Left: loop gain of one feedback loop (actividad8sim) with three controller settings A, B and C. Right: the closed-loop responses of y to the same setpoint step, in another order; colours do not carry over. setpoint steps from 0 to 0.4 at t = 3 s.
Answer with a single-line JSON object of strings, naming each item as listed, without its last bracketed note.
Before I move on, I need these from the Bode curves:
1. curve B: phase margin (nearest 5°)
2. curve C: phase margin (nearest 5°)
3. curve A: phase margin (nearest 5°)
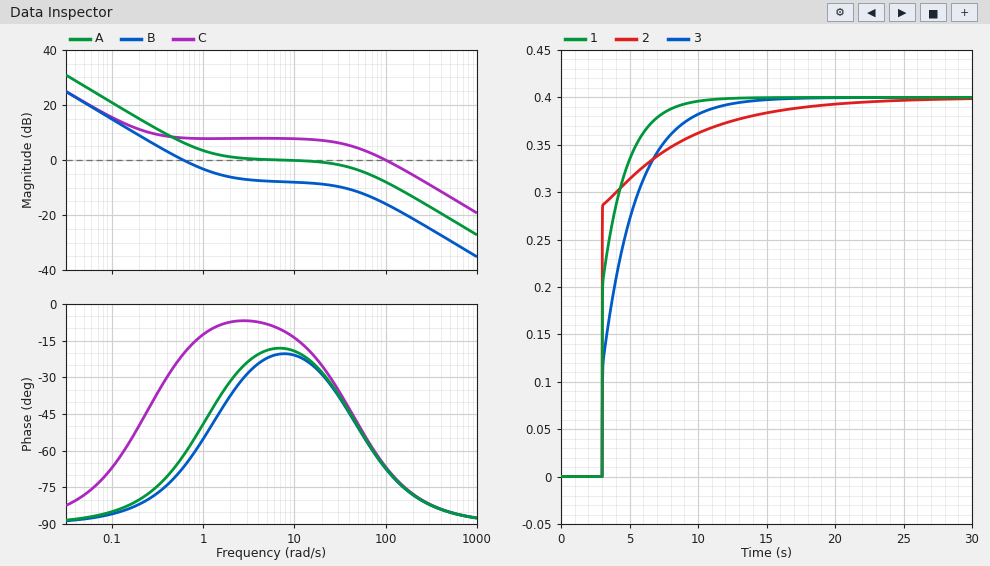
{"curve B: phase margin": "115°", "curve C: phase margin": "115°", "curve A: phase margin": "160°"}
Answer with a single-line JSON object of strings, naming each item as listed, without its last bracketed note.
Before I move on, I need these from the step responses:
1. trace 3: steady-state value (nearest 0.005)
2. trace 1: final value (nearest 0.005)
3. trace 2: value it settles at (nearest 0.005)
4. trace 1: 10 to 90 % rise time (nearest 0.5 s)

{"trace 3: steady-state value": "0.400", "trace 1: final value": "0.400", "trace 2: value it settles at": "0.400", "trace 1: 10 to 90 % rise time": "3.0 s"}
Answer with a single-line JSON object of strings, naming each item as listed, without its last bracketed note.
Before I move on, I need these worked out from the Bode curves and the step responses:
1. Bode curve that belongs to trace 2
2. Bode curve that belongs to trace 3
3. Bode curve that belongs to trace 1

{"Bode curve that belongs to trace 2": "C", "Bode curve that belongs to trace 3": "B", "Bode curve that belongs to trace 1": "A"}
